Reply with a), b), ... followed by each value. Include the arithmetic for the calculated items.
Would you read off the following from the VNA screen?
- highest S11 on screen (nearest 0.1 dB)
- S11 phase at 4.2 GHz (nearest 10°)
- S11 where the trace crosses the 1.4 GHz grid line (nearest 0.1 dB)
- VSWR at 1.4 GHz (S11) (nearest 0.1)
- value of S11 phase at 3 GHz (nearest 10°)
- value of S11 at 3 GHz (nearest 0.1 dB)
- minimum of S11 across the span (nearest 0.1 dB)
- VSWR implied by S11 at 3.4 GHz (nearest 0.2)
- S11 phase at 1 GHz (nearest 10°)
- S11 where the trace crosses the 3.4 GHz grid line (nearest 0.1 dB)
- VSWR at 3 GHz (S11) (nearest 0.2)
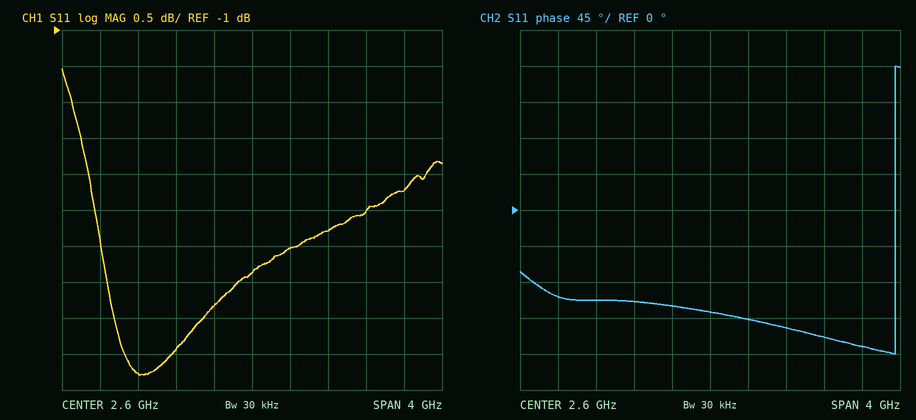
a) -1.5 dB
b) -170°
c) -5.8 dB
d) |Γ| = 10^(-5.8/20) = 0.5129; VSWR = (1 + 0.5129)/(1 − 0.5129) ≈ 3.1
e) -140°
f) -4.0 dB
g) -5.8 dB
h) |Γ| = 10^(-3.8/20) = 0.6457; VSWR = (1 + 0.6457)/(1 − 0.6457) ≈ 4.6
i) -110°
j) -3.8 dB
k) |Γ| = 10^(-4/20) = 0.6310; VSWR = (1 + 0.6310)/(1 − 0.6310) ≈ 4.4
